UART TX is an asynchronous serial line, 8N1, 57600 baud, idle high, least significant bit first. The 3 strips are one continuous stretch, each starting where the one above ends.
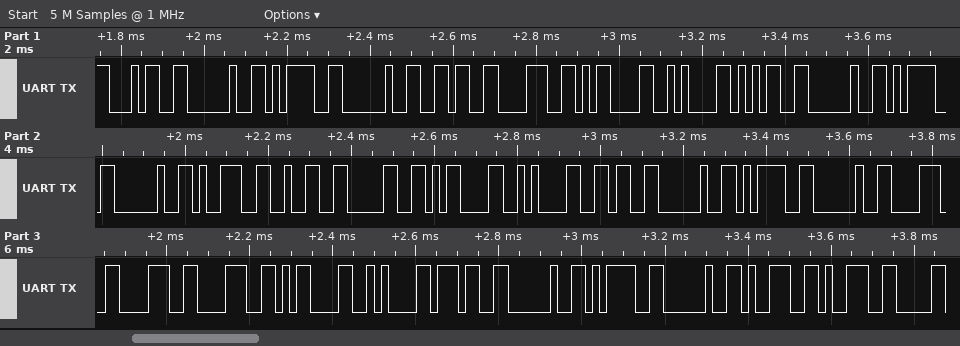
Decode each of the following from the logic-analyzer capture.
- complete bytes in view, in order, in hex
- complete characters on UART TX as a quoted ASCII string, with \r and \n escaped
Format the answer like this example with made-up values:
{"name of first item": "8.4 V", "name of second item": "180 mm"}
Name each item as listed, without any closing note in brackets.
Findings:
{"complete bytes in view, in order, in hex": "0x34 0x20 0x3D 0x20 0x36 0x38 0x0D 0x0A 0x35 0x20 0x3D 0x20 0x39 0x32 0x30 0x0D 0x0A 0x36 0x20 0x3D 0x20 0x38 0x38 0x38 0x0D 0x0A 0x37 0x20 0x3D 0x20 0x39 0x39", "complete characters on UART TX as a quoted ASCII string, with \\r and \\n escaped": "\"4 = 68\\r\\n5 = 920\\r\\n6 = 888\\r\\n7 = 99\""}
